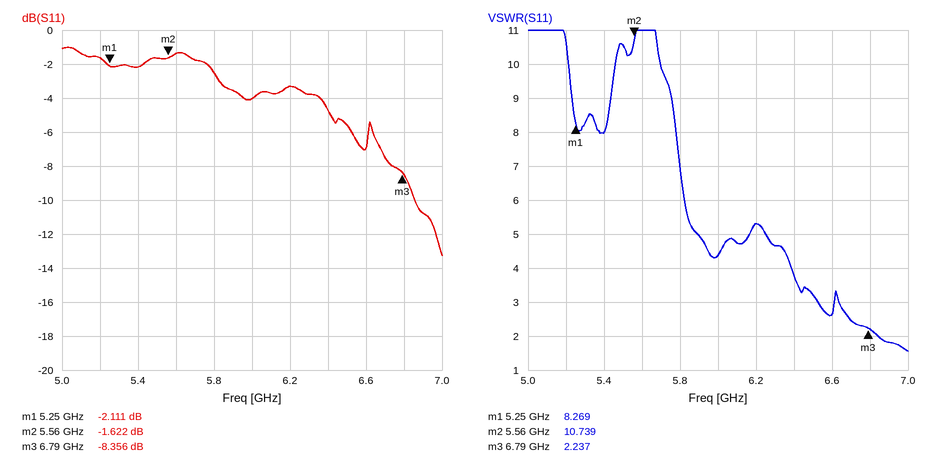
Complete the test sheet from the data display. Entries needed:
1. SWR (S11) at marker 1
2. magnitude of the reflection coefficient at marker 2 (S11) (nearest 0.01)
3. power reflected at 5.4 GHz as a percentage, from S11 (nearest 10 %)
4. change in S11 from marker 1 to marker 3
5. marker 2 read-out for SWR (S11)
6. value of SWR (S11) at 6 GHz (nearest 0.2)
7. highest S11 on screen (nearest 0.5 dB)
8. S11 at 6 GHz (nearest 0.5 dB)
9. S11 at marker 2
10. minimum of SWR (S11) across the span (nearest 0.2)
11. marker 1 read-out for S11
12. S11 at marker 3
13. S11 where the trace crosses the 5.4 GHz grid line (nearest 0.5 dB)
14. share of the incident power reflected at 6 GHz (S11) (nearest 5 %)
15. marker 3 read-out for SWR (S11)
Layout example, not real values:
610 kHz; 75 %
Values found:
8.269; 0.83; 60 %; -6.245 dB; 10.739; 4.4; -1.0 dB; -4.0 dB; -1.622 dB; 1.6; -2.111 dB; -8.356 dB; -2.0 dB; 40 %; 2.237
